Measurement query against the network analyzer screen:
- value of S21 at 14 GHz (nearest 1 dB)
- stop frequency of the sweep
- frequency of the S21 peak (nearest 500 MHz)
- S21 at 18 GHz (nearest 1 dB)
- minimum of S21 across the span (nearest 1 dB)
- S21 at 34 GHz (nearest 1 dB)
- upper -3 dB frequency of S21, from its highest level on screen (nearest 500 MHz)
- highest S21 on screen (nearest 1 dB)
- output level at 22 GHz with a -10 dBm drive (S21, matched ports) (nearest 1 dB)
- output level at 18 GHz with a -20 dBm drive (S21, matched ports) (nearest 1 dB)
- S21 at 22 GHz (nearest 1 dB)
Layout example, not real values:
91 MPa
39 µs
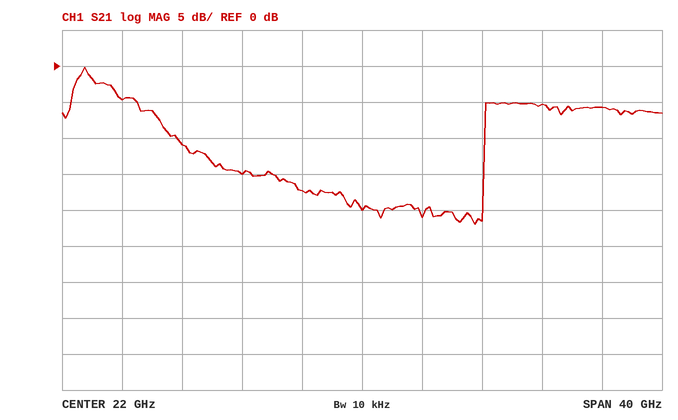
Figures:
-15 dB
42 GHz
3.5 GHz
-17 dB
-22 dB
-5 dB
5.5 GHz
0 dB
-30 dBm
-37 dBm
-20 dB
